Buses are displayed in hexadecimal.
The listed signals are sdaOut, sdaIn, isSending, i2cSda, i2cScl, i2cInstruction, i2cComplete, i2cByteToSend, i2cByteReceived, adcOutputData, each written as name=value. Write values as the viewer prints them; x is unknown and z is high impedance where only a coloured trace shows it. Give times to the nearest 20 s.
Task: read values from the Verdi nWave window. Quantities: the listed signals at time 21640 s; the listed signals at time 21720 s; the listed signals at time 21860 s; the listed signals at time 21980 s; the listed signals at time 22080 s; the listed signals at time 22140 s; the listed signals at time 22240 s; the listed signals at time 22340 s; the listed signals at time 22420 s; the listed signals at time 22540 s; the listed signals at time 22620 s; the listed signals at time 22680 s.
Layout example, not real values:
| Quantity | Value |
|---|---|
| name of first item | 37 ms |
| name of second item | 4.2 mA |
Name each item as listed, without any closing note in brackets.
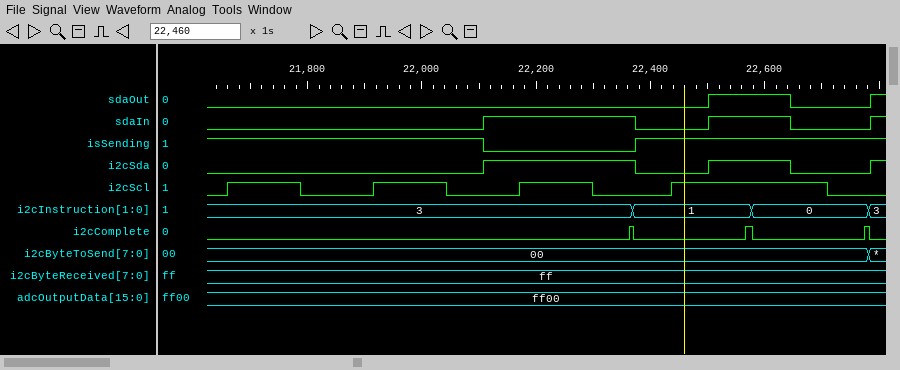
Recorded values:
| Quantity | Value |
|---|---|
| the listed signals at time 21640 s | sdaOut=0, sdaIn=0, isSending=1, i2cSda=0, i2cScl=0, i2cInstruction=3, i2cComplete=0, i2cByteToSend=00, i2cByteReceived=ff, adcOutputData=ff00 |
| the listed signals at time 21720 s | sdaOut=0, sdaIn=0, isSending=1, i2cSda=0, i2cScl=1, i2cInstruction=3, i2cComplete=0, i2cByteToSend=00, i2cByteReceived=ff, adcOutputData=ff00 |
| the listed signals at time 21860 s | sdaOut=0, sdaIn=0, isSending=1, i2cSda=0, i2cScl=0, i2cInstruction=3, i2cComplete=0, i2cByteToSend=00, i2cByteReceived=ff, adcOutputData=ff00 |
| the listed signals at time 21980 s | sdaOut=0, sdaIn=0, isSending=1, i2cSda=0, i2cScl=1, i2cInstruction=3, i2cComplete=0, i2cByteToSend=00, i2cByteReceived=ff, adcOutputData=ff00 |
| the listed signals at time 22080 s | sdaOut=0, sdaIn=0, isSending=1, i2cSda=0, i2cScl=0, i2cInstruction=3, i2cComplete=0, i2cByteToSend=00, i2cByteReceived=ff, adcOutputData=ff00 |
| the listed signals at time 22140 s | sdaOut=0, sdaIn=1, isSending=0, i2cSda=1, i2cScl=0, i2cInstruction=3, i2cComplete=0, i2cByteToSend=00, i2cByteReceived=ff, adcOutputData=ff00 |
| the listed signals at time 22240 s | sdaOut=0, sdaIn=1, isSending=0, i2cSda=1, i2cScl=1, i2cInstruction=3, i2cComplete=0, i2cByteToSend=00, i2cByteReceived=ff, adcOutputData=ff00 |
| the listed signals at time 22340 s | sdaOut=0, sdaIn=1, isSending=0, i2cSda=1, i2cScl=0, i2cInstruction=3, i2cComplete=0, i2cByteToSend=00, i2cByteReceived=ff, adcOutputData=ff00 |
| the listed signals at time 22420 s | sdaOut=0, sdaIn=0, isSending=1, i2cSda=0, i2cScl=0, i2cInstruction=1, i2cComplete=0, i2cByteToSend=00, i2cByteReceived=ff, adcOutputData=ff00 |
| the listed signals at time 22540 s | sdaOut=1, sdaIn=1, isSending=1, i2cSda=1, i2cScl=1, i2cInstruction=1, i2cComplete=0, i2cByteToSend=00, i2cByteReceived=ff, adcOutputData=ff00 |
| the listed signals at time 22620 s | sdaOut=1, sdaIn=1, isSending=1, i2cSda=1, i2cScl=1, i2cInstruction=0, i2cComplete=0, i2cByteToSend=00, i2cByteReceived=ff, adcOutputData=ff00 |
| the listed signals at time 22680 s | sdaOut=0, sdaIn=0, isSending=1, i2cSda=0, i2cScl=1, i2cInstruction=0, i2cComplete=0, i2cByteToSend=00, i2cByteReceived=ff, adcOutputData=ff00 |
